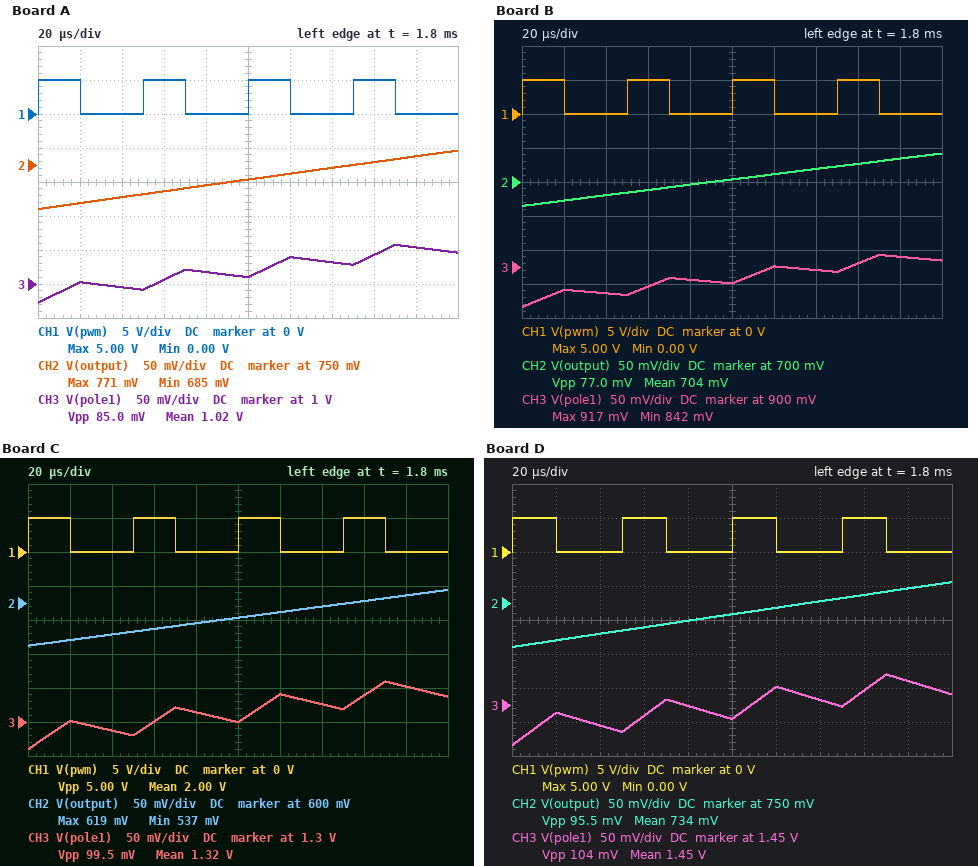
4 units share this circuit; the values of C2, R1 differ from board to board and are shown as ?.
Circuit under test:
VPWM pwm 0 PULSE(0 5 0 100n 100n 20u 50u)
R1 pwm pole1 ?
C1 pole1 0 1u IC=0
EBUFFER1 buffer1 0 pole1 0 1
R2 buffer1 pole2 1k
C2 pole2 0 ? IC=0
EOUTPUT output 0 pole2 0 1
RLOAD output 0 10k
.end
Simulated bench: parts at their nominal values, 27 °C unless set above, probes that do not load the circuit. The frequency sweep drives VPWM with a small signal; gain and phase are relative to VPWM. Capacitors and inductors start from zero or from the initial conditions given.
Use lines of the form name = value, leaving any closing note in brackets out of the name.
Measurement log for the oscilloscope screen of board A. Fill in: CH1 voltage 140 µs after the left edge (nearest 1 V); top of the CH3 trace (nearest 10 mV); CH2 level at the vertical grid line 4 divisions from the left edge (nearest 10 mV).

CH1 voltage 140 µs after the left edge = 0 V
top of the CH3 trace = 1.06 V
CH2 level at the vertical grid line 4 divisions from the left edge = 720 mV
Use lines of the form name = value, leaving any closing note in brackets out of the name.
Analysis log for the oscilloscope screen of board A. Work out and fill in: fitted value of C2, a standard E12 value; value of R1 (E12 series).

fitted value of C2, a standard E12 value = 680 nF
value of R1 = 2.7 kΩ
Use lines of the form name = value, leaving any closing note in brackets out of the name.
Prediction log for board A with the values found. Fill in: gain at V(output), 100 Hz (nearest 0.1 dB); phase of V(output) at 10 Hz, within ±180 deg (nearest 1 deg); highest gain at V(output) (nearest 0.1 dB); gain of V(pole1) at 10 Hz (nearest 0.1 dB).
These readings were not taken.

gain at V(output), 100 Hz = -6.6 dB
phase of V(output) at 10 Hz, within ±180 deg = -12 deg
highest gain at V(output) = 0 dB
gain of V(pole1) at 10 Hz = -0.1 dB
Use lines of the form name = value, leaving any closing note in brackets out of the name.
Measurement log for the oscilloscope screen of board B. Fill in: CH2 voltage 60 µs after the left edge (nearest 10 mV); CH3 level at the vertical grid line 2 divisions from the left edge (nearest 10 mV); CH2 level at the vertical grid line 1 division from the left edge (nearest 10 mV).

CH2 voltage 60 µs after the left edge = 690 mV
CH3 level at the vertical grid line 2 divisions from the left edge = 860 mV
CH2 level at the vertical grid line 1 division from the left edge = 670 mV
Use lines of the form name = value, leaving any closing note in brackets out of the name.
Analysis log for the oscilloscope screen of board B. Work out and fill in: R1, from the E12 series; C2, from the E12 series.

R1, from the E12 series = 3.3 kΩ
C2, from the E12 series = 470 nF
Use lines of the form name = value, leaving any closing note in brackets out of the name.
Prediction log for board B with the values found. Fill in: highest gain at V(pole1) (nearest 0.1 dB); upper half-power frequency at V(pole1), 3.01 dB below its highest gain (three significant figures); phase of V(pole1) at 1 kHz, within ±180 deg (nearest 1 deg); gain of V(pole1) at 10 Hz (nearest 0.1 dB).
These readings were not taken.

highest gain at V(pole1) = 0 dB
upper half-power frequency at V(pole1), 3.01 dB below its highest gain = 48.2 Hz
phase of V(pole1) at 1 kHz, within ±180 deg = -87 deg
gain of V(pole1) at 10 Hz = -0.2 dB
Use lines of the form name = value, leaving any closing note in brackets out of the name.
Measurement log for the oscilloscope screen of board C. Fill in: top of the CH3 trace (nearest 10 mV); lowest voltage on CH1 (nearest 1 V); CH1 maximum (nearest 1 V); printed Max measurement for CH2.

top of the CH3 trace = 1.36 V
lowest voltage on CH1 = 0 V
CH1 maximum = 5 V
printed Max measurement for CH2 = 619 mV
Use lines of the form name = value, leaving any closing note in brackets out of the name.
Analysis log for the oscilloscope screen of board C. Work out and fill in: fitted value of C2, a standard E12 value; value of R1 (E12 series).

fitted value of C2, a standard E12 value = 1.8 µF
value of R1 = 1.8 kΩ
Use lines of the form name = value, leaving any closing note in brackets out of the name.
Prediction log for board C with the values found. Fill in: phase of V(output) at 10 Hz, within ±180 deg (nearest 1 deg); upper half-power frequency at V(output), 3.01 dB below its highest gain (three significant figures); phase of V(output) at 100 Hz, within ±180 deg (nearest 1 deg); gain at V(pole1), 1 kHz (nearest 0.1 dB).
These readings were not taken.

phase of V(output) at 10 Hz, within ±180 deg = -13 deg
upper half-power frequency at V(output), 3.01 dB below its highest gain = 56.9 Hz
phase of V(output) at 100 Hz, within ±180 deg = -97 deg
gain at V(pole1), 1 kHz = -21.1 dB
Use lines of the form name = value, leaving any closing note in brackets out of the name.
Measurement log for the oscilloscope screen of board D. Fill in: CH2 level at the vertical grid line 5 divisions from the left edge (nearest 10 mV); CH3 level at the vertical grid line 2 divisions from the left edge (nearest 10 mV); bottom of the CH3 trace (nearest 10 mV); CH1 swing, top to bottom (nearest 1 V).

CH2 level at the vertical grid line 5 divisions from the left edge = 730 mV
CH3 level at the vertical grid line 2 divisions from the left edge = 1.42 V
bottom of the CH3 trace = 1.39 V
CH1 swing, top to bottom = 5 V
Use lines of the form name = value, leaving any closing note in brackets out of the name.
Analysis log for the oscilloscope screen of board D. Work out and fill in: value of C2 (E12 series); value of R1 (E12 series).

value of C2 = 1.5 µF
value of R1 = 1.5 kΩ
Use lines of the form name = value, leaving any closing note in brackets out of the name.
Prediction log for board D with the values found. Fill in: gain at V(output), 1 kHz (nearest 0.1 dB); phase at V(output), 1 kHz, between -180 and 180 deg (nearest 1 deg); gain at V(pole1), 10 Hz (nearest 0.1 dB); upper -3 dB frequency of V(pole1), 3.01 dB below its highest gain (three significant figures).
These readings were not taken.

gain at V(output), 1 kHz = -39.1 dB
phase at V(output), 1 kHz, between -180 and 180 deg = -168 deg
gain at V(pole1), 10 Hz = 0 dB
upper -3 dB frequency of V(pole1), 3.01 dB below its highest gain = 106 Hz
